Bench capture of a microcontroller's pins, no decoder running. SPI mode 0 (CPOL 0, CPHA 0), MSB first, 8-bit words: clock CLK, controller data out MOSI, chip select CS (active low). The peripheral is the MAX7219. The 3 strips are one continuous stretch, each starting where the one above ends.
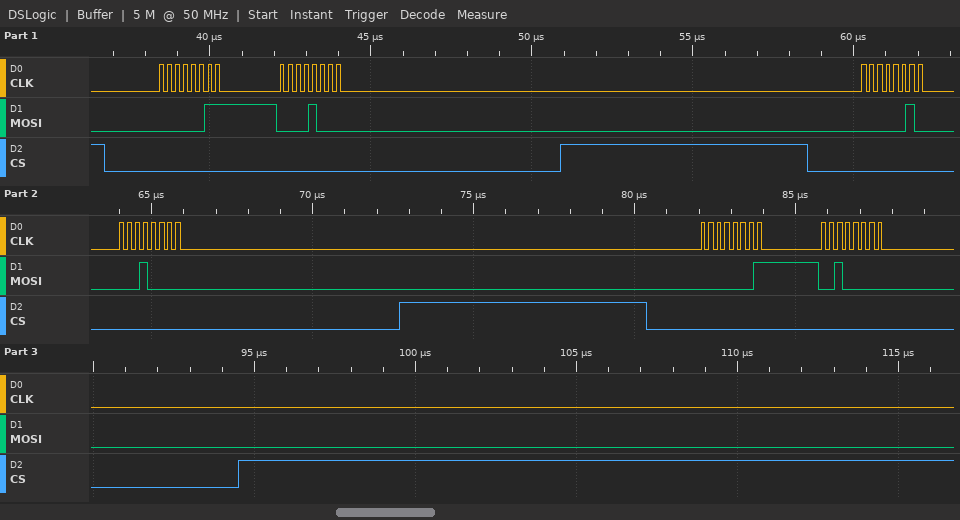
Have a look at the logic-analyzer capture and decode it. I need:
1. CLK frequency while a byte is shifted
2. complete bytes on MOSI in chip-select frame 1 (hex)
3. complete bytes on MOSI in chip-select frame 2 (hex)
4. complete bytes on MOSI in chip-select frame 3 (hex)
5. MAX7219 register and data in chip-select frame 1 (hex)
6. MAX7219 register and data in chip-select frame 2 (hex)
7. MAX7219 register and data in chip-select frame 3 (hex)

4 MHz
03 08
02 10
01 20
register 0x3, data 0x08
register 0x2, data 0x10
register 0x1, data 0x20
